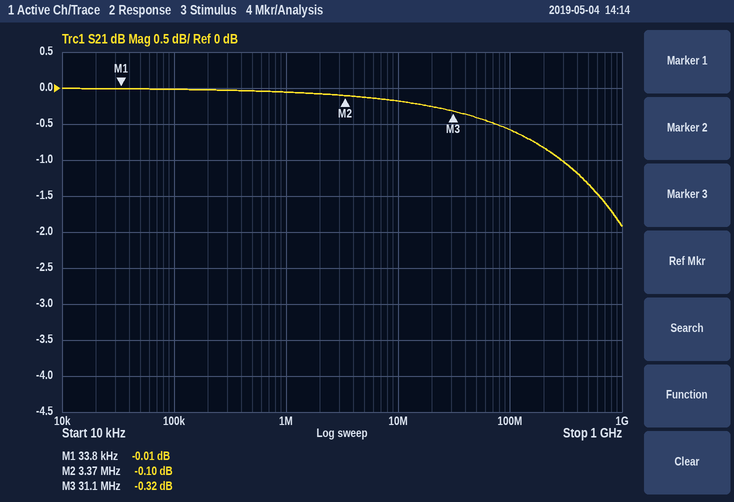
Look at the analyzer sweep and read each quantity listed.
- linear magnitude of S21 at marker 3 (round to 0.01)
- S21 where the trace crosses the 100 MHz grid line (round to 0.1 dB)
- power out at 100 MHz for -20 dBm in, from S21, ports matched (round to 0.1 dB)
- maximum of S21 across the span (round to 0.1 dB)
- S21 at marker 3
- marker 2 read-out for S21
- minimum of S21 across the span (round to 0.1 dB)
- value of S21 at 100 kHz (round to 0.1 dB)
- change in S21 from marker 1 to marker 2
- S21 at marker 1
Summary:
0.96
-0.6 dB
-20.6 dBm
0.0 dB
-0.32 dB
-0.10 dB
-1.9 dB
0.0 dB
-0.09 dB
-0.01 dB
